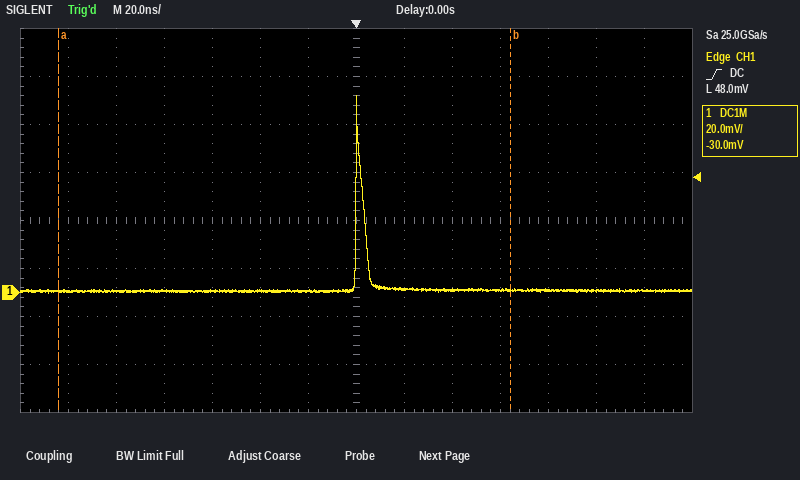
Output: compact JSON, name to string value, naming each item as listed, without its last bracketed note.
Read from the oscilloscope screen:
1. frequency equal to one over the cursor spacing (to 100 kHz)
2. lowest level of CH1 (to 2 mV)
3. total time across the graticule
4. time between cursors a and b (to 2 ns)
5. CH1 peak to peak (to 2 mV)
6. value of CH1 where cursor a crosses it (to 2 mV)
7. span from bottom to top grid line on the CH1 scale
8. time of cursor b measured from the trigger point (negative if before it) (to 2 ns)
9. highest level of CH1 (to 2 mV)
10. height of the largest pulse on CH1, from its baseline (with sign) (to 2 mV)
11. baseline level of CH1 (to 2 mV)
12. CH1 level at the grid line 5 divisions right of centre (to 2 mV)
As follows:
{"frequency equal to one over the cursor spacing": "5.3 MHz", "lowest level of CH1": "0 mV", "total time across the graticule": "280 ns", "time between cursors a and b": "188 ns", "CH1 peak to peak": "82 mV", "value of CH1 where cursor a crosses it": "0 mV", "span from bottom to top grid line on the CH1 scale": "160 mV", "time of cursor b measured from the trigger point (negative if before it)": "+64 ns", "highest level of CH1": "82 mV", "height of the largest pulse on CH1, from its baseline (with sign)": "+82 mV", "baseline level of CH1": "0 mV", "CH1 level at the grid line 5 divisions right of centre": "0 mV"}
